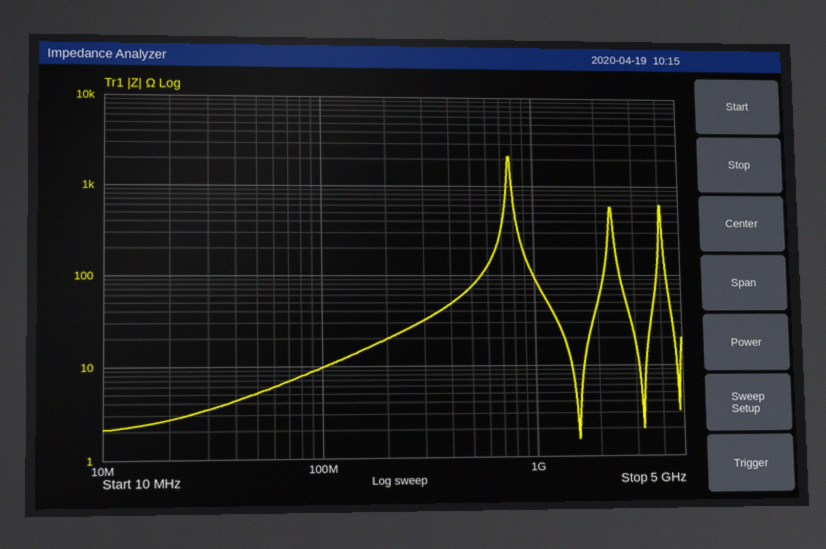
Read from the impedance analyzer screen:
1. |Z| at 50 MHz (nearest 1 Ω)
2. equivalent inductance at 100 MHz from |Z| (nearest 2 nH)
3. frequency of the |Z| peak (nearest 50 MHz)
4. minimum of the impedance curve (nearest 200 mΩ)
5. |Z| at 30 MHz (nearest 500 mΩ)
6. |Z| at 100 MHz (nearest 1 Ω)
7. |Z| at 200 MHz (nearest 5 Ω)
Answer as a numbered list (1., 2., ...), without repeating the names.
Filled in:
1. 5 Ω
2. 16 nH
3. 750 MHz
4. 1.6 Ω
5. 3.5 Ω
6. 10 Ω
7. 20 Ω
